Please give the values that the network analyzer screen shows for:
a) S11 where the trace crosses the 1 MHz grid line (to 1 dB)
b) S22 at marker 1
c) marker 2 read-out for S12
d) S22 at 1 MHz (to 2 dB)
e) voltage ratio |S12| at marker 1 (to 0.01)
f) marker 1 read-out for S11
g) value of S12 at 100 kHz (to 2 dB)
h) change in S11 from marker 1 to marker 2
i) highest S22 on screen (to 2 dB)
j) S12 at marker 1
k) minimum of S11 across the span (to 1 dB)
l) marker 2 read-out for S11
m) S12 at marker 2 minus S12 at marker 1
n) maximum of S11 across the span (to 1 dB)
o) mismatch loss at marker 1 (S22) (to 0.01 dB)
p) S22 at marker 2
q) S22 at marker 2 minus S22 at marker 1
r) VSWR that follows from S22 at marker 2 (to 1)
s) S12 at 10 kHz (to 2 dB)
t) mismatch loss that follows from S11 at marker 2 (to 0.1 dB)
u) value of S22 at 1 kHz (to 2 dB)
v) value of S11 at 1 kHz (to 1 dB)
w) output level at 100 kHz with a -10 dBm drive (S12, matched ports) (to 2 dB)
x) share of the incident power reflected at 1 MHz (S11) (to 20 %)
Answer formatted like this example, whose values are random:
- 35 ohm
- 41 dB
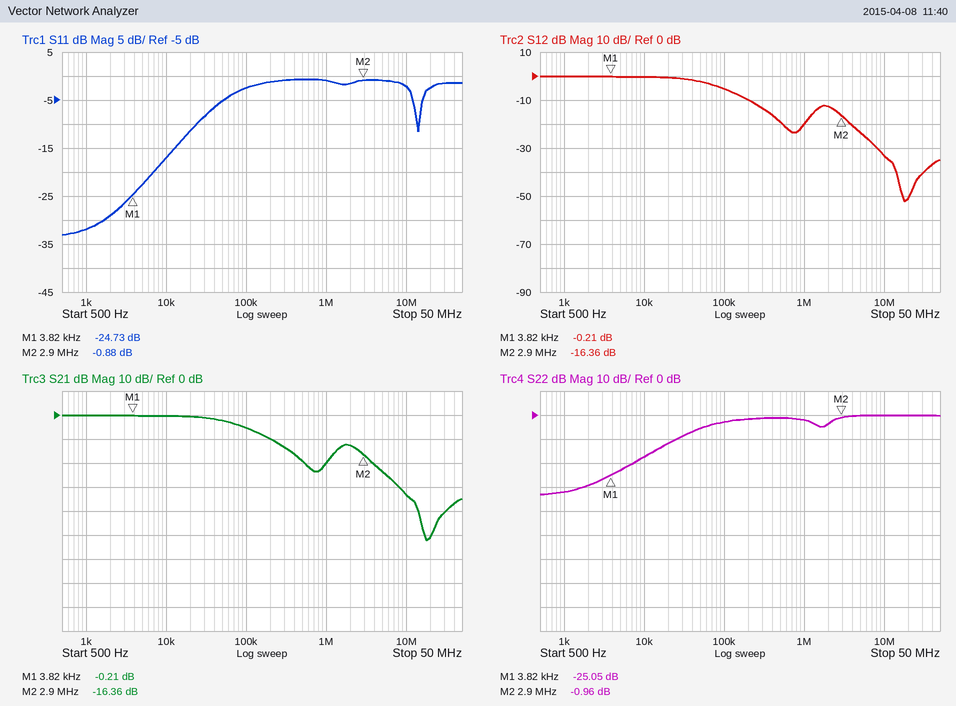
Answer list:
- -1 dB
- -25.05 dB
- -16.36 dB
- -2 dB
- 0.98
- -24.73 dB
- -6 dB
- 23.85 dB
- 0 dB
- -0.21 dB
- -33 dB
- -0.88 dB
- -16.15 dB
- -1 dB
- 0.01 dB
- -0.96 dB
- 24.09 dB
- 18
- 0 dB
- 7.4 dB
- -32 dB
- -32 dB
- -16 dBm
- 80 %
